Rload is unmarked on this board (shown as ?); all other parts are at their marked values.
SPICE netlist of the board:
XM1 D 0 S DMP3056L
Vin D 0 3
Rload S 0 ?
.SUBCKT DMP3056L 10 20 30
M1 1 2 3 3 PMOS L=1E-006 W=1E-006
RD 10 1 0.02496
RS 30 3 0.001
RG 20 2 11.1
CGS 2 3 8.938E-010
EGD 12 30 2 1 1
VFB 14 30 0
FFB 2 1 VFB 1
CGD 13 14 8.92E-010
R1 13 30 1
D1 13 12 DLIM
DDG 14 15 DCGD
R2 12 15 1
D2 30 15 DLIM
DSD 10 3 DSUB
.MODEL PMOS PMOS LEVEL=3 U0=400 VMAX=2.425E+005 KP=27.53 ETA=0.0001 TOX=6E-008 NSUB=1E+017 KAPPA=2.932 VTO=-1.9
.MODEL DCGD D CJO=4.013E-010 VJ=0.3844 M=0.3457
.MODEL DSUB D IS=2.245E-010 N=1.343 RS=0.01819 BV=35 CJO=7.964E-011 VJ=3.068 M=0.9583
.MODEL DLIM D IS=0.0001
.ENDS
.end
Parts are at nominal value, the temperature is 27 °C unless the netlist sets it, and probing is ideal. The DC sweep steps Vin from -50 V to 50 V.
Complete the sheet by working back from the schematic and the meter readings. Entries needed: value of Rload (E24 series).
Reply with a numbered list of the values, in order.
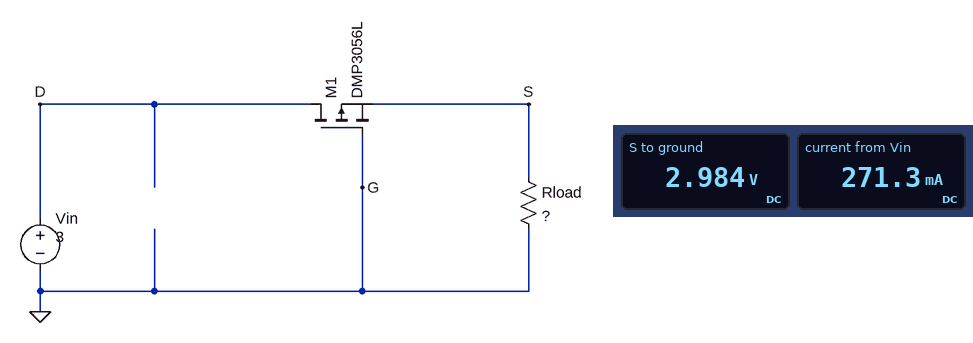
1. 11 Ω
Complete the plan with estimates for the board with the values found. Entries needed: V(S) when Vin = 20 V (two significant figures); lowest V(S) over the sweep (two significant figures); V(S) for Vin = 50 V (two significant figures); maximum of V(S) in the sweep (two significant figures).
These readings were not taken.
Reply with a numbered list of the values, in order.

1. 20 V
2. -15 V
3. 50 V
4. 50 V
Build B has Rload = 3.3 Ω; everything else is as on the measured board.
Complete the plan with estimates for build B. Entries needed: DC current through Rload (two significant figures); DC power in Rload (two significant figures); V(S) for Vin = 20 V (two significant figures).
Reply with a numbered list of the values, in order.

1. 890 mA
2. 2.6 W
3. 20 V
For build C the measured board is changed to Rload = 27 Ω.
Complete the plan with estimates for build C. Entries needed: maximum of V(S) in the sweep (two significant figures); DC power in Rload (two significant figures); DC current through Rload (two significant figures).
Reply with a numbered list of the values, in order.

1. 50 V
2. 330 mW
3. 110 mA
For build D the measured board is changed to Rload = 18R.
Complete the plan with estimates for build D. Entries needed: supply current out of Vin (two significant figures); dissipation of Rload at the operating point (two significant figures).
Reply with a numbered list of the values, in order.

1. 170 mA
2. 500 mW
